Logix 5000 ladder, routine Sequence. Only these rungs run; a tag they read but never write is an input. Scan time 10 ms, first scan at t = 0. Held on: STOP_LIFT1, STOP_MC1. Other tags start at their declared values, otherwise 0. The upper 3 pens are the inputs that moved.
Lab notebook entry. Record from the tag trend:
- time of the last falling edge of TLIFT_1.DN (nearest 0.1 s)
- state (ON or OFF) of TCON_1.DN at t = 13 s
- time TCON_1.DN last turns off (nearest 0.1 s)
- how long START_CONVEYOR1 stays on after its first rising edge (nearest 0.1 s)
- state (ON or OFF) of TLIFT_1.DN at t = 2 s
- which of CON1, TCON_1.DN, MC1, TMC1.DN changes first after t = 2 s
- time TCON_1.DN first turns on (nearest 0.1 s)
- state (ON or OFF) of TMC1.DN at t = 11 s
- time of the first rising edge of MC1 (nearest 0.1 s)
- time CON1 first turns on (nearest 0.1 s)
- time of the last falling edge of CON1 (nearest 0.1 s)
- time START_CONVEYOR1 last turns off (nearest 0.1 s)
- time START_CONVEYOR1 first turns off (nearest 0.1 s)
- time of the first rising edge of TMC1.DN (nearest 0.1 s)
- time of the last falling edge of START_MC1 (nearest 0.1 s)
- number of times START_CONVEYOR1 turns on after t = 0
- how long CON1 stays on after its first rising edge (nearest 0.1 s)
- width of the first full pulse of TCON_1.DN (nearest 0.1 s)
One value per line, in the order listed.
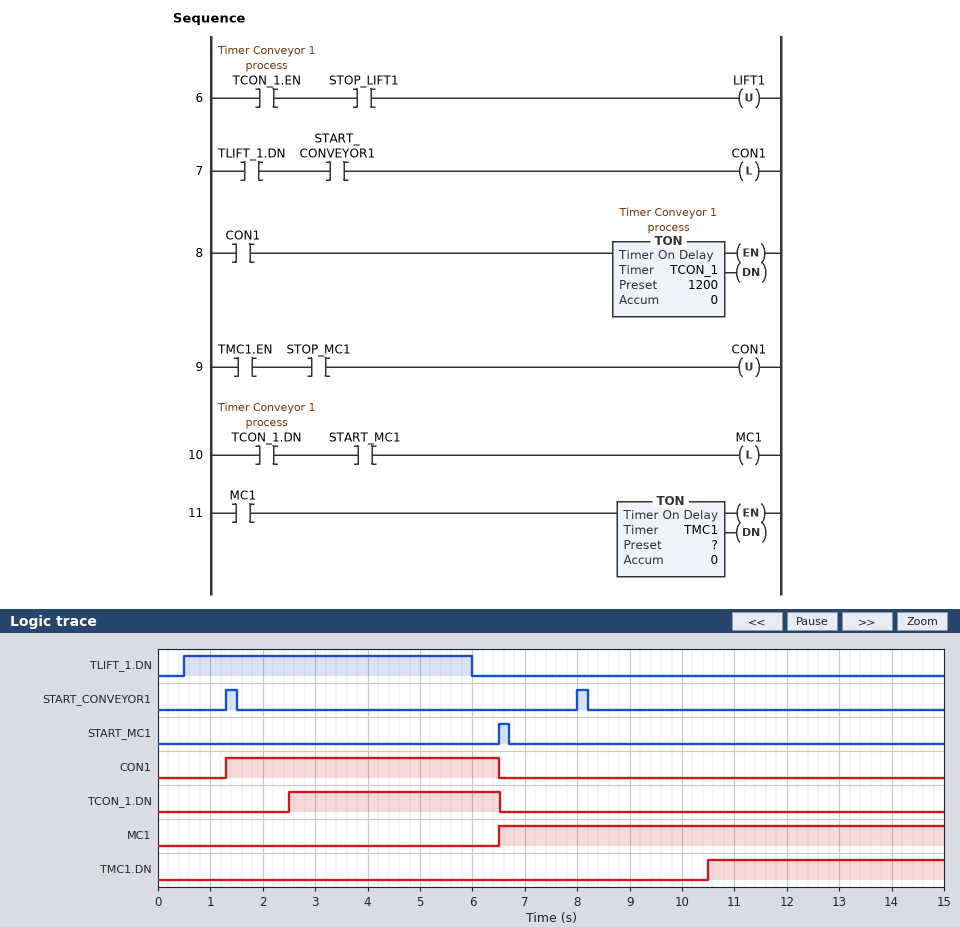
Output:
6.0 s
OFF
6.5 s
0.2 s
ON
TCON_1.DN
2.5 s
ON
6.5 s
1.3 s
6.5 s
8.2 s
1.5 s
10.5 s
6.7 s
2
5.2 s
4.0 s
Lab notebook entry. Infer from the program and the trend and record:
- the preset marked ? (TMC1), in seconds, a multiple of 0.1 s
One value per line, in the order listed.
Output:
4.0 s
